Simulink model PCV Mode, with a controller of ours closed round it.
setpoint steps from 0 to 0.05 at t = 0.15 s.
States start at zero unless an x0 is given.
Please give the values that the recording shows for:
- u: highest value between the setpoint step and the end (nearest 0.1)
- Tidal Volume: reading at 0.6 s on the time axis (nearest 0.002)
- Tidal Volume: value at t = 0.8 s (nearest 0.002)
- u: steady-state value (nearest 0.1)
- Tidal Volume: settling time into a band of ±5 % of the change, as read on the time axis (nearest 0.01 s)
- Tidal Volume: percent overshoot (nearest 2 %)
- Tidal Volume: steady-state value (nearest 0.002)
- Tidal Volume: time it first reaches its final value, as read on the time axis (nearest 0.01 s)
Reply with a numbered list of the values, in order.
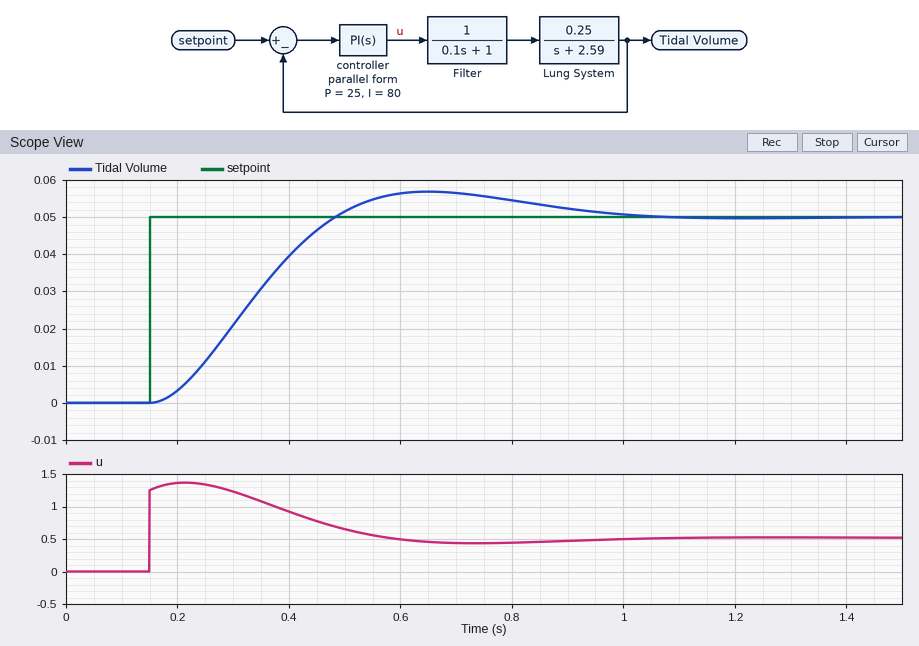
1. 1.4
2. 0.056
3. 0.054
4. 0.5
5. 0.89 s
6. 14 %
7. 0.050
8. 0.48 s
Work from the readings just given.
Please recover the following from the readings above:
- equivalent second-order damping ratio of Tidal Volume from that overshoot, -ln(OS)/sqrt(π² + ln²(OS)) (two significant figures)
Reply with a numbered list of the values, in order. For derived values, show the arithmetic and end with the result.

1. ln(0.14) = -1.966; 1.966 / sqrt(9.870 + 3.866) = 0.53
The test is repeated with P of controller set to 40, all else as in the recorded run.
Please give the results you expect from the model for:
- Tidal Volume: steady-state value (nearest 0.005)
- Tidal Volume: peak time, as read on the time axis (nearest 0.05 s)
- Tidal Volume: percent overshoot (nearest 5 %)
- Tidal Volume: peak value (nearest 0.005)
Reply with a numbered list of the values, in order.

1. 0.050
2. 0.50 s
3. 10 %
4. 0.055
